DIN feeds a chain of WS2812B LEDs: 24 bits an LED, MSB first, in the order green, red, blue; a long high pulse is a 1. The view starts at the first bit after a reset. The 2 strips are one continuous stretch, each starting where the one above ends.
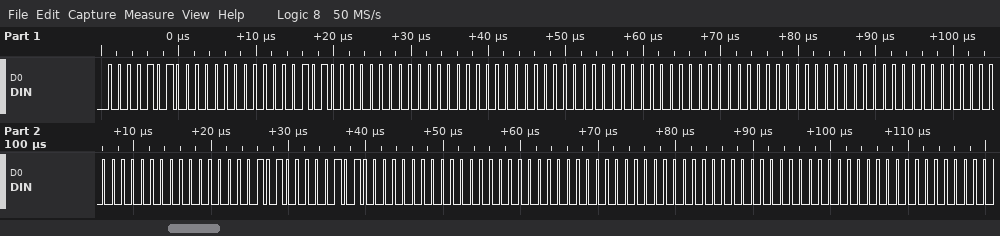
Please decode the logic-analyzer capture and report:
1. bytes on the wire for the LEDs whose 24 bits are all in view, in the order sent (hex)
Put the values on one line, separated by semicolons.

0A 00 0A 00 00 00 00 00 00 00 00 00 00 0A 0A 00 00 00 00 00 00
